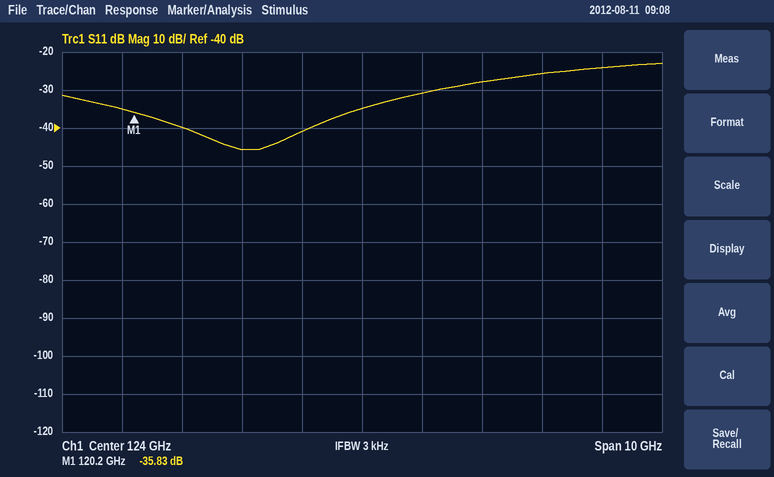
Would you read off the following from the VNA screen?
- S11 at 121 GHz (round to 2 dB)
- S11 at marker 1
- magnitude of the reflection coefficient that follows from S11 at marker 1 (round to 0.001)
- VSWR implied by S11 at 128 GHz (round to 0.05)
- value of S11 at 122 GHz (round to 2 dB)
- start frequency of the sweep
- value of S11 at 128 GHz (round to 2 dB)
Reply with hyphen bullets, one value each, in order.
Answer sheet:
- -40 dB
- -35.83 dB
- 0.016
- 1.15
- -46 dB
- 119 GHz
- -24 dB
